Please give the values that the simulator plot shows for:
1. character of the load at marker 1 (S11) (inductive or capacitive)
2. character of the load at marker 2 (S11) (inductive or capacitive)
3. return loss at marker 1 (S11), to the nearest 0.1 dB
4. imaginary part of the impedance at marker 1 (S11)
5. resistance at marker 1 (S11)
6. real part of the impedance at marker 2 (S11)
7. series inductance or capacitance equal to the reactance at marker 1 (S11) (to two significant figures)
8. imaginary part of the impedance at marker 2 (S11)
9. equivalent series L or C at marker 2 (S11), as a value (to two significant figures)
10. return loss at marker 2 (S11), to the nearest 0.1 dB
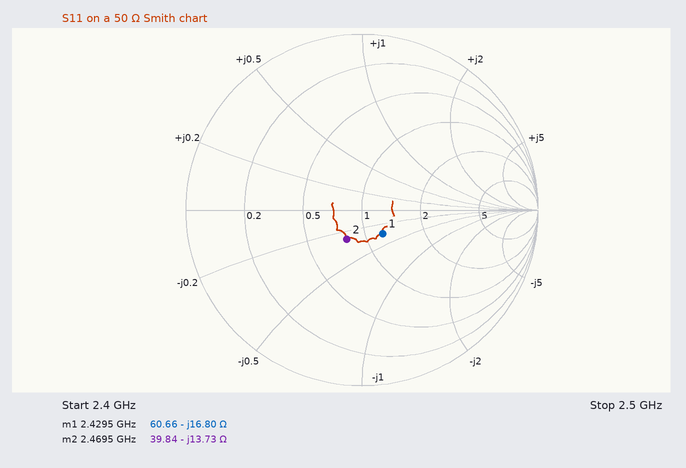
capacitive
capacitive
15.0 dB
-16.80 Ω
60.66 Ω
39.84 Ω
3.9 pF
-13.73 Ω
4.7 pF
14.5 dB
